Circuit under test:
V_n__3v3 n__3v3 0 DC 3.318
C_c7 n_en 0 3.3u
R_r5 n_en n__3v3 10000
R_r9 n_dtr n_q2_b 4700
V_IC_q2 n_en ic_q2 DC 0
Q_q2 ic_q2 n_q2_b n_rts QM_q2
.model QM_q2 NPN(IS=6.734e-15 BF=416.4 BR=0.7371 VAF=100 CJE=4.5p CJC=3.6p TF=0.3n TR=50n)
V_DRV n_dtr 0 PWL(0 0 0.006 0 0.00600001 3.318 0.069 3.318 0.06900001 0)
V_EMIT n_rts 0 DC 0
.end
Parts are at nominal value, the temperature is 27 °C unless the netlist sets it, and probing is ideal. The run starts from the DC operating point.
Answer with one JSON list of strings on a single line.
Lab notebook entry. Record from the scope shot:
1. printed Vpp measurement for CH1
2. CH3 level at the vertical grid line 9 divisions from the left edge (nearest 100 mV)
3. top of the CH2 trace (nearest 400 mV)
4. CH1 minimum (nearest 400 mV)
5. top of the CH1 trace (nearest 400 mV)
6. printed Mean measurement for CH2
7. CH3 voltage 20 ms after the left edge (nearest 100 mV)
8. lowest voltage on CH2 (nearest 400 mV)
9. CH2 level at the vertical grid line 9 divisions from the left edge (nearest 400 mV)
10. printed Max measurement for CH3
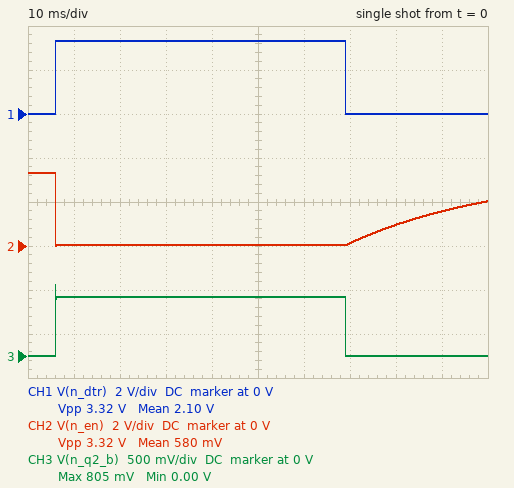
["3.32 V", "0 V", "3.2 V", "0 V", "3.2 V", "580 mV", "700 mV", "0 V", "1.6 V", "805 mV"]
